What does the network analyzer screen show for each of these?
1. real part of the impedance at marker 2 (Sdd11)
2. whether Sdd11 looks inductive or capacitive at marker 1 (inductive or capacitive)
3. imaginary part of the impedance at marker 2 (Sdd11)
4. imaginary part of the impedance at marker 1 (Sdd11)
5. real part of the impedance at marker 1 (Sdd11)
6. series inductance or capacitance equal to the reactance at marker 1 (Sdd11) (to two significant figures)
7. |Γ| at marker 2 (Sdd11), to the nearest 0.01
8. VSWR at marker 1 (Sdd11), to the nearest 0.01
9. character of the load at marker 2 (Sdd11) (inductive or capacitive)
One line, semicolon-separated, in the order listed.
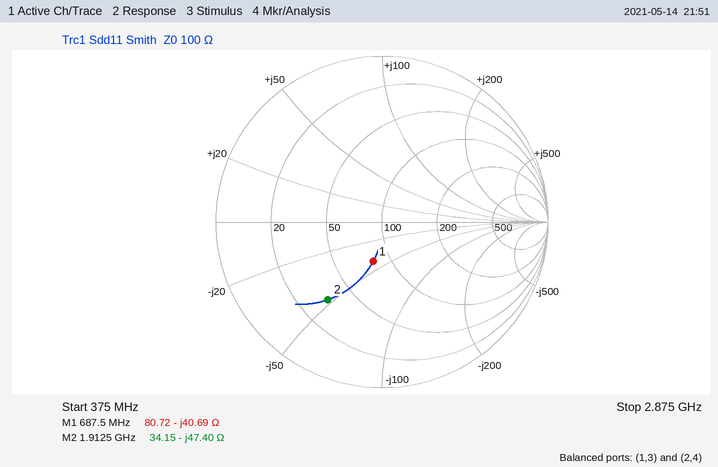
34.15 Ω; capacitive; -47.40 Ω; -40.69 Ω; 80.72 Ω; 5.7 pF; 0.57; 1.64; capacitive
